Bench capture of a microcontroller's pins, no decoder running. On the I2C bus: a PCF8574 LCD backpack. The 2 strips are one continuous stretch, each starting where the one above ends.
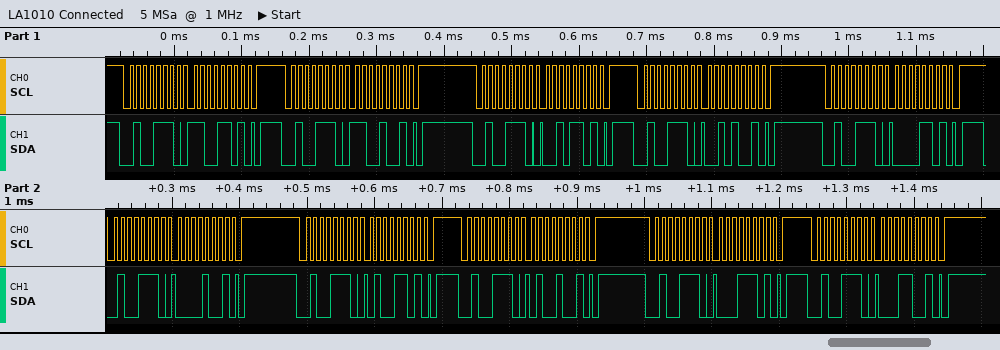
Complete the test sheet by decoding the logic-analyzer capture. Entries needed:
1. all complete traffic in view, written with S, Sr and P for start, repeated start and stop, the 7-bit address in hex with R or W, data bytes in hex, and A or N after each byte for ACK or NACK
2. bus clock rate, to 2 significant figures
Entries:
S 27W A CD A P S 27W A C9 A P S 27W A 2D A P S 27W A 29 A P S 27W A 0D A P S 27W A 09 A P S 27W A 4D A P S 27W A 49 A P S 27W A 1D A P S 27W A 19 A P
100 kHz
